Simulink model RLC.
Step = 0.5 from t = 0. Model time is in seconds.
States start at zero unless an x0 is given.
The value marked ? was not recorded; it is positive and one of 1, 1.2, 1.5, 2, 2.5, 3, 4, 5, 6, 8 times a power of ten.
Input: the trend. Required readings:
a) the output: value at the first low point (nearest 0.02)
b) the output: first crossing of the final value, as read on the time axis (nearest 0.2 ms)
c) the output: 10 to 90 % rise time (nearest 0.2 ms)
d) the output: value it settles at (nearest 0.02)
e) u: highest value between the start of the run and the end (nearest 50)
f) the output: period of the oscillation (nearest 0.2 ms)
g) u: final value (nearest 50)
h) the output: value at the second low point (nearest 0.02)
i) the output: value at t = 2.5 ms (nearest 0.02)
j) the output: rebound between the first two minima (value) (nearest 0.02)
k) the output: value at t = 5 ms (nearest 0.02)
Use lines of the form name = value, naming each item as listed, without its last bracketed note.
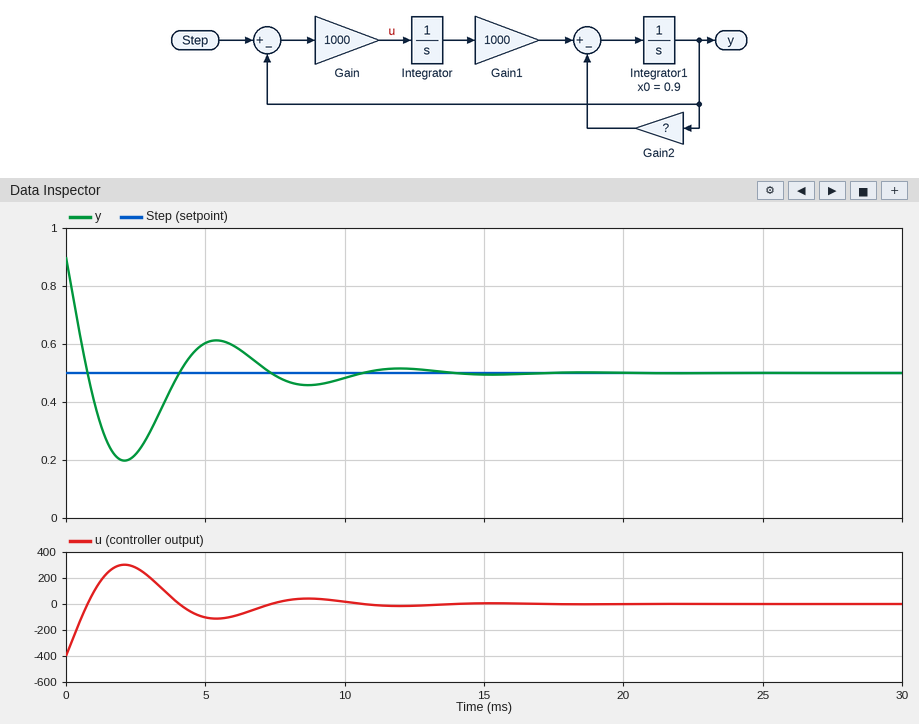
the output: value at the first low point = 0.20
the output: first crossing of the final value, as read on the time axis = 0.8 ms
the output: 10 to 90 % rise time = 0.6 ms
the output: value it settles at = 0.50
u: highest value between the start of the run and the end = 300
the output: period of the oscillation = 6.6 ms
u: final value = 0
the output: value at the second low point = 0.46
the output: value at t = 2.5 ms = 0.22
the output: rebound between the first two minima (value) = 0.62
the output: value at t = 5 ms = 0.60
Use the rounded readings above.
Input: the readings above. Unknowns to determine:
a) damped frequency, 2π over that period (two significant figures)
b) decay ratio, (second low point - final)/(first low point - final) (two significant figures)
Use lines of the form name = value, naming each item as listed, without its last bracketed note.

damped frequency, 2π over that period = 0.95 rad/ms
decay ratio, (second low point - final)/(first low point - final) = 0.13
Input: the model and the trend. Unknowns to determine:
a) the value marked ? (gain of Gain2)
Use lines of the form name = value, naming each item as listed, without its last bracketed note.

the value marked ? = 600
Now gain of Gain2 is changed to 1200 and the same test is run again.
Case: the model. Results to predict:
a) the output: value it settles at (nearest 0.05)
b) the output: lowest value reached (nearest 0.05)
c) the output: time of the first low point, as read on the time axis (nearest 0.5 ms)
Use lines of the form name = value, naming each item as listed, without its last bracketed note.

the output: value it settles at = 0.50
the output: lowest value reached = 0.15
the output: time of the first low point, as read on the time axis = 1.5 ms
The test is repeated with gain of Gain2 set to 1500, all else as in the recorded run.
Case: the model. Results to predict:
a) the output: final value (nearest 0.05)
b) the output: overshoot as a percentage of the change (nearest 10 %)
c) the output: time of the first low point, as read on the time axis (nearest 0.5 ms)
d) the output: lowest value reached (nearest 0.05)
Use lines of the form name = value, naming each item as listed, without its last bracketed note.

the output: final value = 0.50
the output: overshoot as a percentage of the change = 90 %
the output: time of the first low point, as read on the time axis = 1.5 ms
the output: lowest value reached = 0.15
